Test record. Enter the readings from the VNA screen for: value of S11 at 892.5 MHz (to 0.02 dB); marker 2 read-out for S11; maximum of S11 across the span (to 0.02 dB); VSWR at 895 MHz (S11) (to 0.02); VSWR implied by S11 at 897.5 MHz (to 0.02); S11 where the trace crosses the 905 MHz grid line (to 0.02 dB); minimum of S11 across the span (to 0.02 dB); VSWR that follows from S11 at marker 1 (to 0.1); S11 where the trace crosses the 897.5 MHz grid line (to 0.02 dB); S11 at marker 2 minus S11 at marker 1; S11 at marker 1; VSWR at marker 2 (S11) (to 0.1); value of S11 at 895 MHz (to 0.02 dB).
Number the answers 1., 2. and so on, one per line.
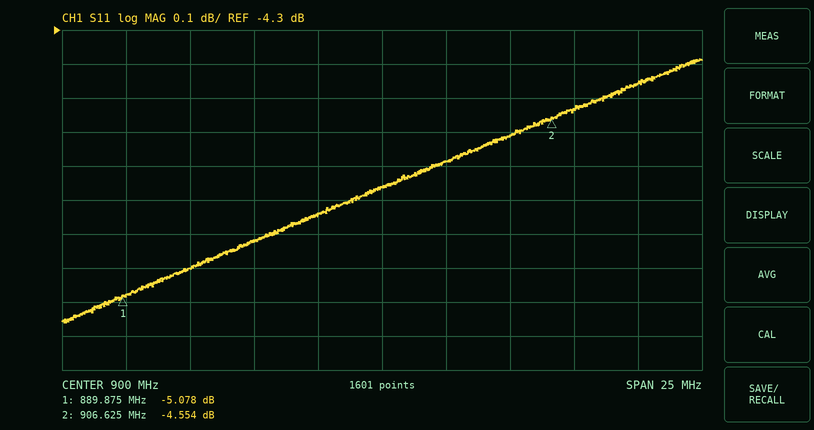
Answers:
1. -5.00 dB
2. -4.554 dB
3. -4.38 dB
4. 3.62
5. 3.68
6. -4.62 dB
7. -5.16 dB
8. 3.5
9. -4.84 dB
10. 0.524 dB
11. -5.078 dB
12. 3.9
13. -4.92 dB
